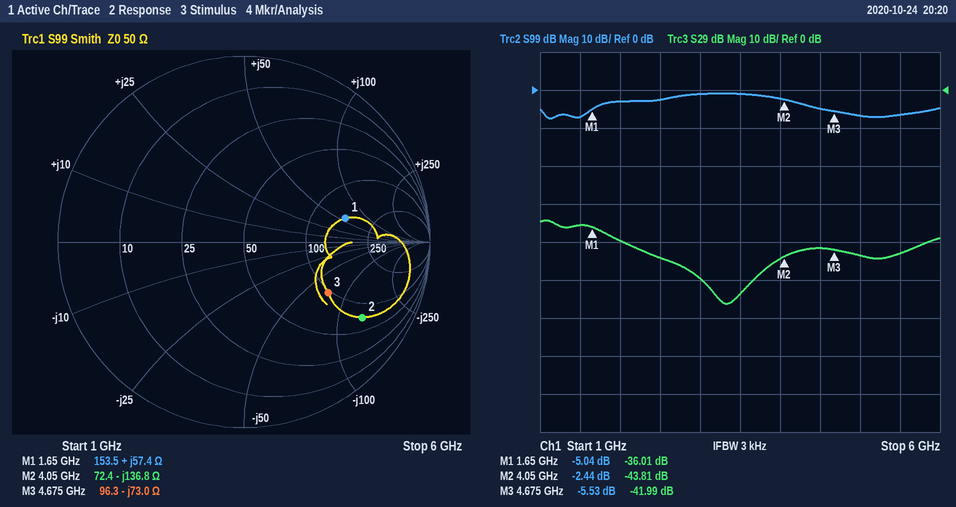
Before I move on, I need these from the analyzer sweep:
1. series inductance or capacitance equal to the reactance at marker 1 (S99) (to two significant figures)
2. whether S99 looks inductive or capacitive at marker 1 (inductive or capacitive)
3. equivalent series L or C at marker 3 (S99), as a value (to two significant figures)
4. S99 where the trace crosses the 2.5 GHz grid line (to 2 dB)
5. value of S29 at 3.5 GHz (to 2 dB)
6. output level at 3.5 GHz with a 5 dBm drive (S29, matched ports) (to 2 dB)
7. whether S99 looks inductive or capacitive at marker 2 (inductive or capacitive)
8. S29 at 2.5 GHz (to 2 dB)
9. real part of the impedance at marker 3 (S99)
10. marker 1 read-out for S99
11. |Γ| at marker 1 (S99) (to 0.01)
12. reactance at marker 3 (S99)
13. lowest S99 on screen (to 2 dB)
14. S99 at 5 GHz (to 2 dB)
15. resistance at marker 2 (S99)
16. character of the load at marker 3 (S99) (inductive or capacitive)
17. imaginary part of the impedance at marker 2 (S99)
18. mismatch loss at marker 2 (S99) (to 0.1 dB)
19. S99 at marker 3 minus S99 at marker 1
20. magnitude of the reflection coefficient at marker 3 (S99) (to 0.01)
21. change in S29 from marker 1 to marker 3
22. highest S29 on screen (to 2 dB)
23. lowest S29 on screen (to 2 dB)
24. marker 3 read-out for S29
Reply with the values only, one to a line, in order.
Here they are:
5.5 nH
inductive
470 fF
-2 dB
-54 dB
-48 dBm
capacitive
-44 dB
96.3 Ω
-5.04 dB
0.56
-73.0 Ω
-8 dB
-6 dB
72.4 Ω
capacitive
-136.8 Ω
3.7 dB
-0.49 dB
0.53
-5.98 dB
-34 dB
-56 dB
-41.99 dB
